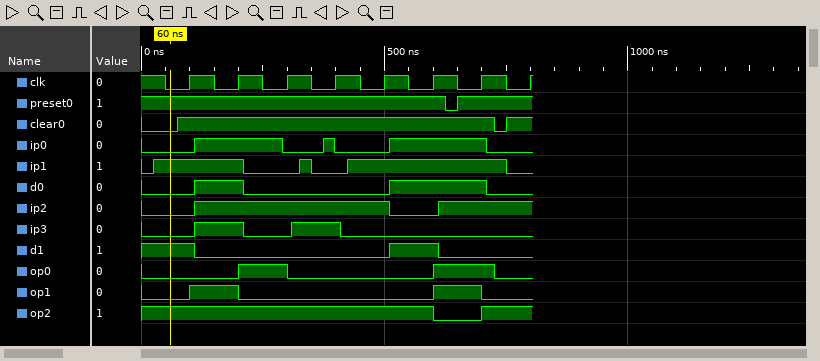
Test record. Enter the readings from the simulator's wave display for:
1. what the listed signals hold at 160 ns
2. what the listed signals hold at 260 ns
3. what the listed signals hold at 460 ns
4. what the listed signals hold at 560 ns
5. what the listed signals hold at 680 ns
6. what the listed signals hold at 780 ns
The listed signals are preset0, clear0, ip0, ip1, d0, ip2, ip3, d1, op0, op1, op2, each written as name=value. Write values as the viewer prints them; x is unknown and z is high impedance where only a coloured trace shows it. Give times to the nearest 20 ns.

preset0=1, clear0=1, ip0=1, ip1=1, d0=1, ip2=1, ip3=1, d1=0, op0=0, op1=1, op2=1
preset0=1, clear0=1, ip0=1, ip1=0, d0=0, ip2=1, ip3=0, d1=0, op0=1, op1=0, op2=1
preset0=1, clear0=1, ip0=0, ip1=1, d0=0, ip2=1, ip3=0, d1=0, op0=0, op1=0, op2=1
preset0=1, clear0=1, ip0=1, ip1=1, d0=1, ip2=0, ip3=0, d1=1, op0=0, op1=0, op2=1
preset0=1, clear0=1, ip0=1, ip1=1, d0=1, ip2=1, ip3=0, d1=0, op0=1, op1=1, op2=0
preset0=1, clear0=1, ip0=0, ip1=0, d0=0, ip2=1, ip3=0, d1=0, op0=0, op1=0, op2=1
